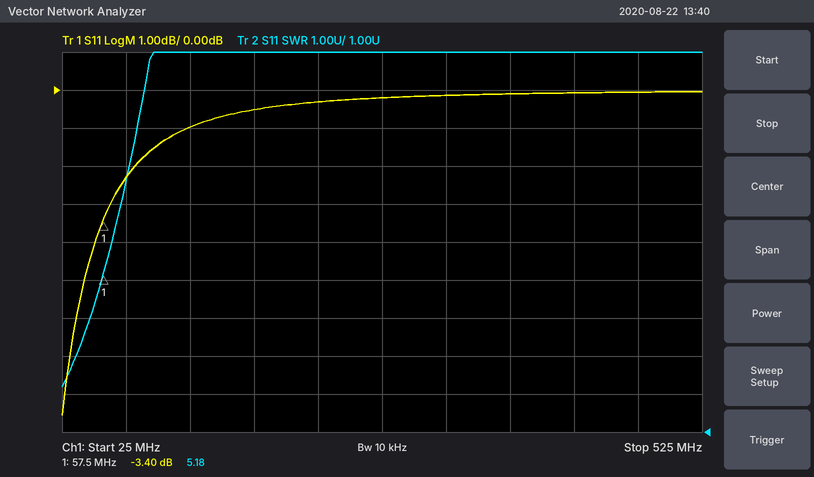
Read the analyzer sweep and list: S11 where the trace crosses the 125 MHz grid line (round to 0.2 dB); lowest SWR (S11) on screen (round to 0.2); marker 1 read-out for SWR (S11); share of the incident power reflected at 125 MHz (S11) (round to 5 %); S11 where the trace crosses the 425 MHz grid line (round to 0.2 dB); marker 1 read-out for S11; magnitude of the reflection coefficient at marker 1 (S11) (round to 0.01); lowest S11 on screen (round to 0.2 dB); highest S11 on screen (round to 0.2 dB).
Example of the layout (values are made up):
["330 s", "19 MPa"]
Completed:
["-1.0 dB", "2.2", "5.18", "80 %", "0.0 dB", "-3.40 dB", "0.68", "-8.6 dB", "0.0 dB"]
